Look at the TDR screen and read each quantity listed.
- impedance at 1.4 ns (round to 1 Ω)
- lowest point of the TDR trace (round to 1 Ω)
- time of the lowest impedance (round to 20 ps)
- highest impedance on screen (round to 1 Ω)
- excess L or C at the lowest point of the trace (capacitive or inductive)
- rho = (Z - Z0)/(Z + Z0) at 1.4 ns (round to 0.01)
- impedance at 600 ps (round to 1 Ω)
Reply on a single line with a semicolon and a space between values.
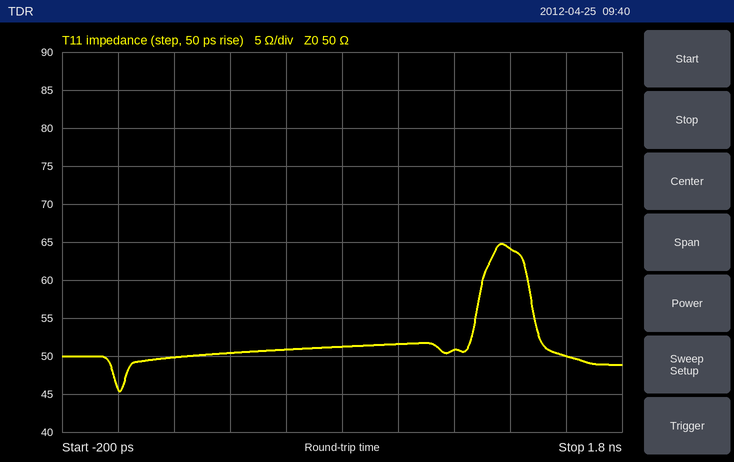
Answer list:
64 Ω; 45 Ω; 0 ps; 65 Ω; capacitive; +0.12; 51 Ω
